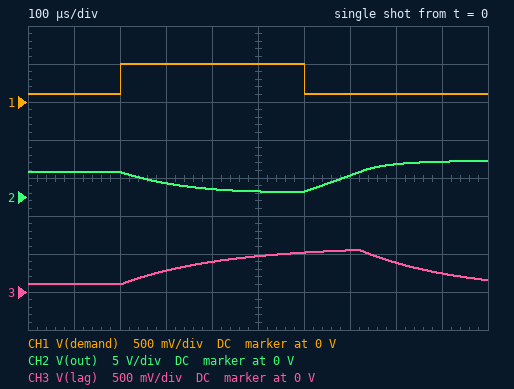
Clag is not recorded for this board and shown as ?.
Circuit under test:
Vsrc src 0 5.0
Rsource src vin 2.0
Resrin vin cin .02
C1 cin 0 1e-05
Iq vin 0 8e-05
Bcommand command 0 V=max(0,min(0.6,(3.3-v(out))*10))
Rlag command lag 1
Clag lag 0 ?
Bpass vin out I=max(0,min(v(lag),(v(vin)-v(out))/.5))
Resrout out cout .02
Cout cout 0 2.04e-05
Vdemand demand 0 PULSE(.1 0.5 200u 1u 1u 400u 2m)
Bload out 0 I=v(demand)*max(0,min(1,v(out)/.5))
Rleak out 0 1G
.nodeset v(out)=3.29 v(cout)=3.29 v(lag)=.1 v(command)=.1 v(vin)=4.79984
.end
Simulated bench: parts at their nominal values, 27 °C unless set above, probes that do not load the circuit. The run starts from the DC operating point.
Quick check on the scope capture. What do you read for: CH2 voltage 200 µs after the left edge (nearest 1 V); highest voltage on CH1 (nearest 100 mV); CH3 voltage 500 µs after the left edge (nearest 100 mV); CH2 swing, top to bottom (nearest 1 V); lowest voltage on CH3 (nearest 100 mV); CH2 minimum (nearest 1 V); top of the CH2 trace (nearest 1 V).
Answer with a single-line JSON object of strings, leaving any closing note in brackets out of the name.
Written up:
{"CH2 voltage 200 µs after the left edge": "3 V", "highest voltage on CH1": "500 mV", "CH3 voltage 500 µs after the left edge": "500 mV", "CH2 swing, top to bottom": "4 V", "lowest voltage on CH3": "100 mV", "CH2 minimum": "1 V", "top of the CH2 trace": "5 V"}
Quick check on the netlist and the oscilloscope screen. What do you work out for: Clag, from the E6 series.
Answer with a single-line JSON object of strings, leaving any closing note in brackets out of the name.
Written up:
{"Clag, from the E6 series": "220 µF"}
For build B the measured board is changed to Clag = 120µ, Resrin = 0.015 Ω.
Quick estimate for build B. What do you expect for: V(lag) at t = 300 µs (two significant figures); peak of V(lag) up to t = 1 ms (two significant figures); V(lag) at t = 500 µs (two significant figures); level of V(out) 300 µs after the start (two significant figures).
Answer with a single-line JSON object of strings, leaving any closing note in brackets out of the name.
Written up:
{"V(lag) at t = 300 µs": "380 mV", "peak of V(lag) up to t = 1 ms": "590 mV", "V(lag) at t = 500 µs": "560 mV", "level of V(out) 300 µs after the start": "2.1 V"}
